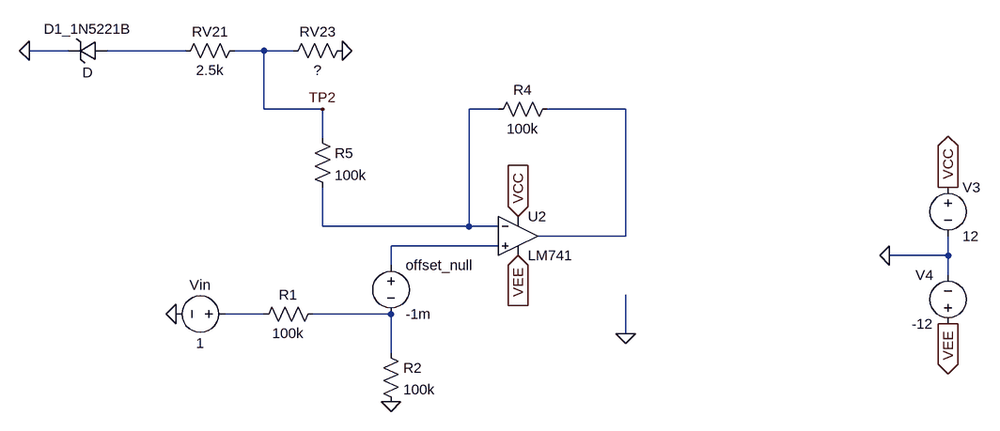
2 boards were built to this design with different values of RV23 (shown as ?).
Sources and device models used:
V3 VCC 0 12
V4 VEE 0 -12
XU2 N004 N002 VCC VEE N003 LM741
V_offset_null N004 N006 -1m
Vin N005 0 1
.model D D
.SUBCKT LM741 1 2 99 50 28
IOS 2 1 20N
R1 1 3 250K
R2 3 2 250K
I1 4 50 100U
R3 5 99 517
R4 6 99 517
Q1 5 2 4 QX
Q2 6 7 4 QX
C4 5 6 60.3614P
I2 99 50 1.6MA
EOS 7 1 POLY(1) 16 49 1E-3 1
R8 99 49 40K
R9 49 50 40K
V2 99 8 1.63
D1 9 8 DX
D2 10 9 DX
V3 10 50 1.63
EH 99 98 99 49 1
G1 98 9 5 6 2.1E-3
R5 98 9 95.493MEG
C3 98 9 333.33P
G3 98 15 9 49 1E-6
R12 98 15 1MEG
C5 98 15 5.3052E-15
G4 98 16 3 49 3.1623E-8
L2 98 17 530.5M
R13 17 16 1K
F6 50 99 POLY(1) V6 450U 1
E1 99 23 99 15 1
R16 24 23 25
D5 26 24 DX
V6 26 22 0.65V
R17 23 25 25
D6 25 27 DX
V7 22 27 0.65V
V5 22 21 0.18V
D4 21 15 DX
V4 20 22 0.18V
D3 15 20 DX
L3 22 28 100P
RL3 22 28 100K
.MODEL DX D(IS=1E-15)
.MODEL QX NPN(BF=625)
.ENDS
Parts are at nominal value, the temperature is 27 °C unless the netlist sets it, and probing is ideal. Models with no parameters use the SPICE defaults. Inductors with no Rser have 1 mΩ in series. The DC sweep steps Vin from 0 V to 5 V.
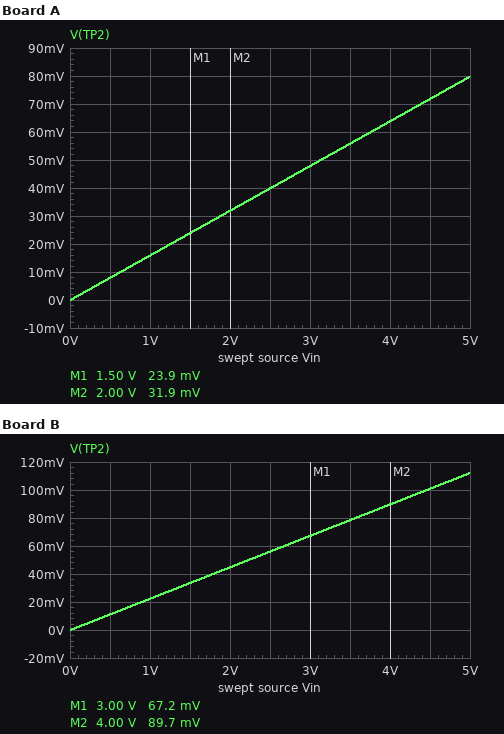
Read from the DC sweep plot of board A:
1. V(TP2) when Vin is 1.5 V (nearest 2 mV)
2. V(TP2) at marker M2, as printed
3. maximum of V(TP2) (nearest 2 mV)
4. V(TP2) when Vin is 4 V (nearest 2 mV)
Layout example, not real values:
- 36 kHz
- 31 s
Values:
- 24 mV
- 31.9 mV
- 80 mV
- 64 mV
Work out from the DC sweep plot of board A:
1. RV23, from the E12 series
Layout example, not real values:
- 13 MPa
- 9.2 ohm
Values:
- 3.3 kΩ
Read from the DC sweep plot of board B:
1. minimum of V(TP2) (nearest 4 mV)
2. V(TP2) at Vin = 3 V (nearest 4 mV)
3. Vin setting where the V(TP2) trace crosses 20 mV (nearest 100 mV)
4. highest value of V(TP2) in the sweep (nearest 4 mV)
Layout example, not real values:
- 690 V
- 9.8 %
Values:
- 0 V
- 68 mV
- 900 mV
- 112 mV
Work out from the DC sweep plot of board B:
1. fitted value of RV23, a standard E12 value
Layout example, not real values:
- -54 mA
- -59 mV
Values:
- 4.7 kΩ
